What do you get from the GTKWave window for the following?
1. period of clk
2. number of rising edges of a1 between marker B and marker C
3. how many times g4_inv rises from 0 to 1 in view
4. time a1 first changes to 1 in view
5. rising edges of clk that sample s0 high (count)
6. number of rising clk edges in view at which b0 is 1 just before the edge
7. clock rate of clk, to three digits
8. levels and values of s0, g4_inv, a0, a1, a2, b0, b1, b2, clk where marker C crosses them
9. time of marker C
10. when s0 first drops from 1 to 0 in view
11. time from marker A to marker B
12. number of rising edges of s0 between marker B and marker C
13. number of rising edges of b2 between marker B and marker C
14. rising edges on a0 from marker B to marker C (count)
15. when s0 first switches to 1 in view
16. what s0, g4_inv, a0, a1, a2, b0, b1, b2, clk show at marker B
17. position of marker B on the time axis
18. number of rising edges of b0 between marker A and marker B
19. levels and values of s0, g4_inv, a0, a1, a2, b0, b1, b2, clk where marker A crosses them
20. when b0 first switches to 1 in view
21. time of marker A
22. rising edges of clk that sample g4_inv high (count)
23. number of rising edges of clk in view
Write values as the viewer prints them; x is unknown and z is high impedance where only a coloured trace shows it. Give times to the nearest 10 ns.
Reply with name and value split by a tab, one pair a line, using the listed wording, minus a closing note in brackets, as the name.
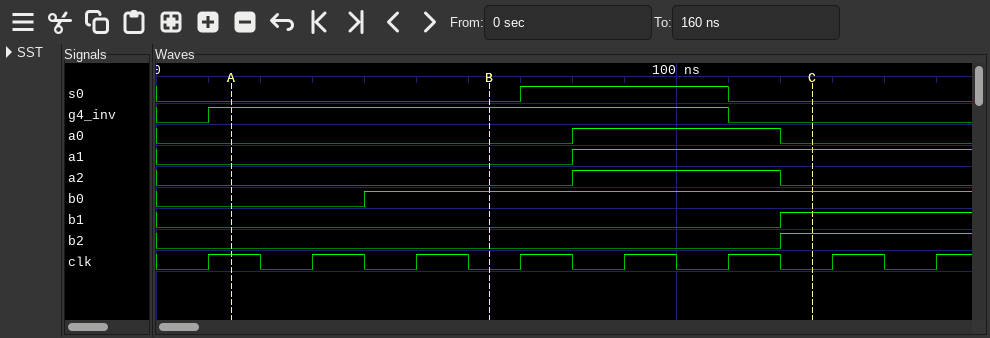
period of clk	20 ns
number of rising edges of a1 between marker B and marker C	1
how many times g4_inv rises from 0 to 1 in view	1
time a1 first changes to 1 in view	80 ns
rising edges of clk that sample s0 high	2
number of rising clk edges in view at which b0 is 1 just before the edge	6
clock rate of clk, to three digits	50.0 MHz
levels and values of s0, g4_inv, a0, a1, a2, b0, b1, b2, clk where marker C crosses them	s0=0, g4_inv=0, a0=0, a1=1, a2=0, b0=1, b1=1, b2=1, clk=0
time of marker C	130 ns
when s0 first drops from 1 to 0 in view	110 ns
time from marker A to marker B	50 ns
number of rising edges of s0 between marker B and marker C	1
number of rising edges of b2 between marker B and marker C	1
rising edges on a0 from marker B to marker C	1
when s0 first switches to 1 in view	70 ns
what s0, g4_inv, a0, a1, a2, b0, b1, b2, clk show at marker B	s0=0, g4_inv=1, a0=0, a1=0, a2=0, b0=1, b1=0, b2=0, clk=0
position of marker B on the time axis	60 ns
number of rising edges of b0 between marker A and marker B	1
levels and values of s0, g4_inv, a0, a1, a2, b0, b1, b2, clk where marker A crosses them	s0=0, g4_inv=1, a0=0, a1=0, a2=0, b0=0, b1=0, b2=0, clk=1
when b0 first switches to 1 in view	40 ns
time of marker A	10 ns
rising edges of clk that sample g4_inv high	5
number of rising edges of clk in view	8
